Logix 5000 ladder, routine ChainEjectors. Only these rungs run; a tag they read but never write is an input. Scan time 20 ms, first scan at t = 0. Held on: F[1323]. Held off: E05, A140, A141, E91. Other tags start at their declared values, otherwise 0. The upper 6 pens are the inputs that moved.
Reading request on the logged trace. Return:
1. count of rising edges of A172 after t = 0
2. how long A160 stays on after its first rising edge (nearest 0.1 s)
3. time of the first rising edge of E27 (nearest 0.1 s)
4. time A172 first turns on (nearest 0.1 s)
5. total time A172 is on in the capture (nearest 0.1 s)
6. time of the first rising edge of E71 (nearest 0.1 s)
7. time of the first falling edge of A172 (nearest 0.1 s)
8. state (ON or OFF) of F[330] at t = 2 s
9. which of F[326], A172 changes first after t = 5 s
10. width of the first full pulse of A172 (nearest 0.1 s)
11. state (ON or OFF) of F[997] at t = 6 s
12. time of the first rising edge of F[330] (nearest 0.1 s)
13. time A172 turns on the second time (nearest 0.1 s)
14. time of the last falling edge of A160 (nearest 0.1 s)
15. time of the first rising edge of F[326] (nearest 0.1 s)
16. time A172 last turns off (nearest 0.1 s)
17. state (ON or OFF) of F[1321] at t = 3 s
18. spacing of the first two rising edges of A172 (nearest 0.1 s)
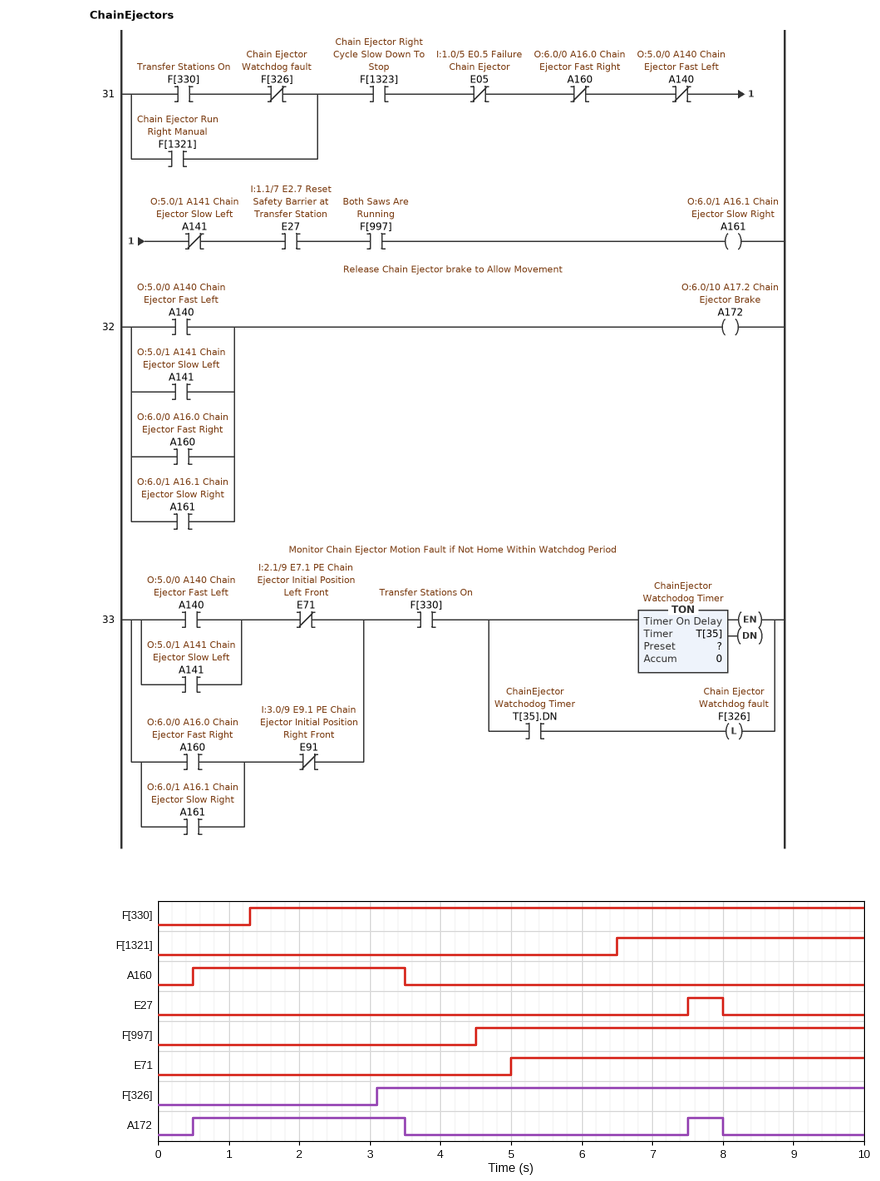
2
3.0 s
7.5 s
0.5 s
3.5 s
5.0 s
3.5 s
ON
A172
3.0 s
ON
1.3 s
7.5 s
3.5 s
3.1 s
8.0 s
OFF
7.0 s
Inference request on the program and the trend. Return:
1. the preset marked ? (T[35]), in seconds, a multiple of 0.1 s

1.8 s
